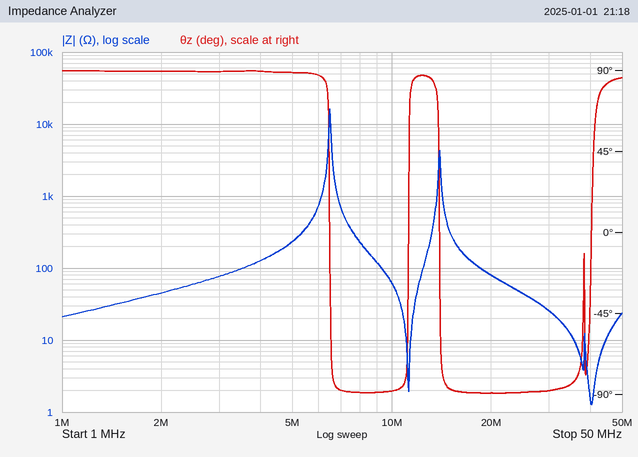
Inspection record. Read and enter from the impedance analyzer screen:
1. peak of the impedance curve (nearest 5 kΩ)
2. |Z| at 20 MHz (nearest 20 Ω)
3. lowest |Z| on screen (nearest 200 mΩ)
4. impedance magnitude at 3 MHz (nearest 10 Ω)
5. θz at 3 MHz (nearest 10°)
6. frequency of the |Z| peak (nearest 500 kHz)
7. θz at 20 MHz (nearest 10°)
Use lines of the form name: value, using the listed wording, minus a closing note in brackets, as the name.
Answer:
peak of the impedance curve: 15 kΩ
|Z| at 20 MHz: 80 Ω
lowest |Z| on screen: 1.2 Ω
impedance magnitude at 3 MHz: 80 Ω
θz at 3 MHz: 90°
frequency of the |Z| peak: 6.5 MHz
θz at 20 MHz: -90°
